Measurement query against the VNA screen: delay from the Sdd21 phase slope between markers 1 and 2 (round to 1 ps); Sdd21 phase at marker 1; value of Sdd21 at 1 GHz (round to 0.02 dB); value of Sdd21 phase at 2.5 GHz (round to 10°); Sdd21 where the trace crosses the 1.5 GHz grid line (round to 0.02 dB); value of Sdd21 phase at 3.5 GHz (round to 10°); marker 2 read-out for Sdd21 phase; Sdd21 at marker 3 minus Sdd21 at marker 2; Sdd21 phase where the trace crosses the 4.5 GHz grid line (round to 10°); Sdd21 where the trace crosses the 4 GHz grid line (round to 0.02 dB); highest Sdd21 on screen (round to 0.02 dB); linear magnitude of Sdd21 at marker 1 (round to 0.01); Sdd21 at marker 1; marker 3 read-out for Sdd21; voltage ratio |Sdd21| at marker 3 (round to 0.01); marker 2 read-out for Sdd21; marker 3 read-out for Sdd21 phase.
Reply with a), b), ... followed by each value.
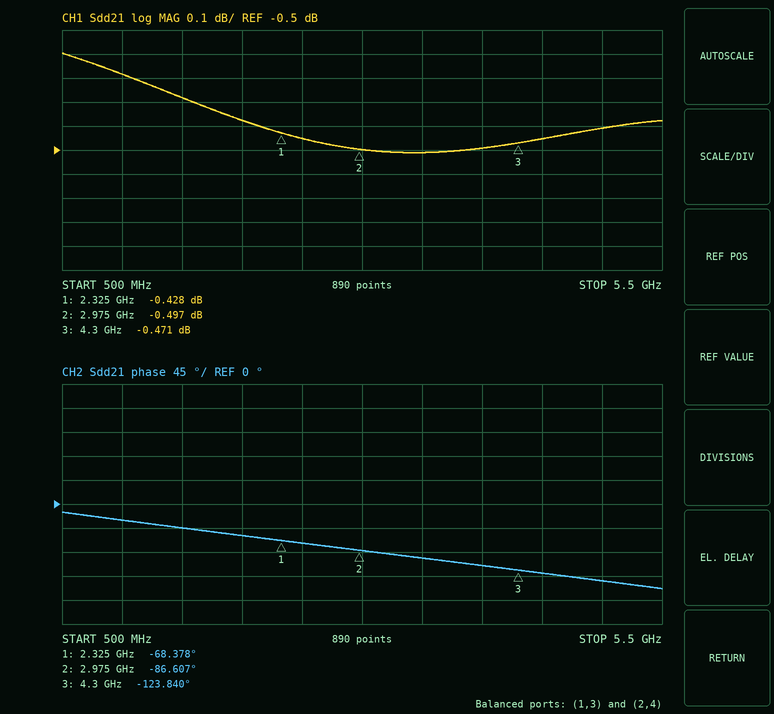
a) 78 ps
b) -68.378°
c) -0.18 dB
d) -70°
e) -0.28 dB
f) -100°
g) -86.607°
h) 0.026 dB
i) -130°
j) -0.50 dB
k) -0.10 dB
l) 0.95
m) -0.428 dB
n) -0.471 dB
o) 0.95
p) -0.497 dB
q) -123.840°
